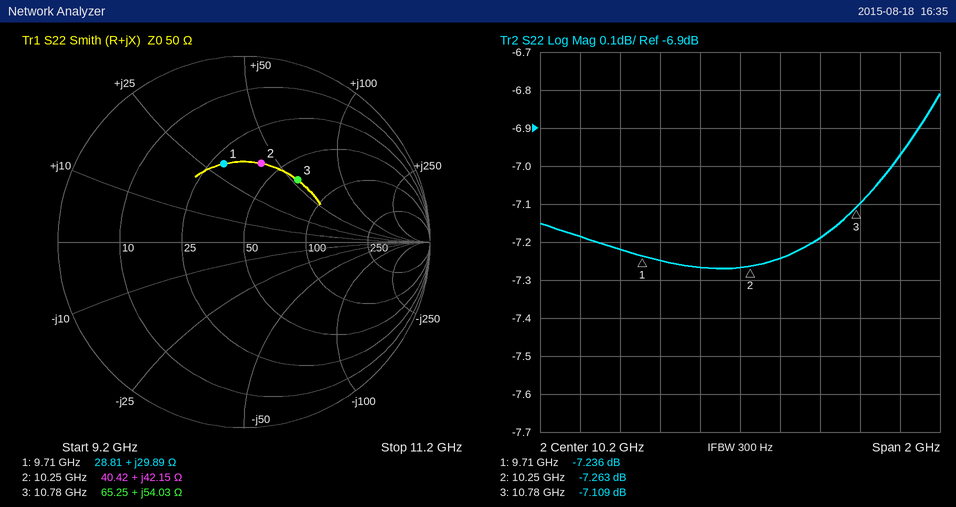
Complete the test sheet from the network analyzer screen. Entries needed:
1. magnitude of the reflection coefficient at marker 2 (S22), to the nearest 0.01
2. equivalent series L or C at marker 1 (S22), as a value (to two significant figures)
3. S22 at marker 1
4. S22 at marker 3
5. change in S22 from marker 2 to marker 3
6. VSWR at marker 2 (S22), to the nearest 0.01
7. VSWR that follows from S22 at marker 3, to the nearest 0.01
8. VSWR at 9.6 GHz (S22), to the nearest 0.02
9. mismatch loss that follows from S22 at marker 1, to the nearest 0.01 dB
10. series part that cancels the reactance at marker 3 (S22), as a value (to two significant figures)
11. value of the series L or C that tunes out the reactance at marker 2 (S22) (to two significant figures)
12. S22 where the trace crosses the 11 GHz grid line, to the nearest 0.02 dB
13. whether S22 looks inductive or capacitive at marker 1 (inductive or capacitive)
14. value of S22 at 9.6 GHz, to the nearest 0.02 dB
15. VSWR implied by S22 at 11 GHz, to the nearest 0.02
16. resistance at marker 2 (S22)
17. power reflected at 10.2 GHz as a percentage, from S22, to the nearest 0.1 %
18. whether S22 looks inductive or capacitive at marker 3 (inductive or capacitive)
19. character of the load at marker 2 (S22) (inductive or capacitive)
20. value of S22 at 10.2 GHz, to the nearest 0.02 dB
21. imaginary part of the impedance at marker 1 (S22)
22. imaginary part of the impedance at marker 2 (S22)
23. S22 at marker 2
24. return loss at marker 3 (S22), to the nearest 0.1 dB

0.43
490 pH
-7.236 dB
-7.109 dB
0.154 dB
2.53
2.58
2.54
0.91 dB
270 fF
370 fF
-6.98 dB
inductive
-7.22 dB
2.62
40.42 Ω
18.8 %
inductive
inductive
-7.26 dB
+29.89 Ω
+42.15 Ω
-7.263 dB
7.1 dB
